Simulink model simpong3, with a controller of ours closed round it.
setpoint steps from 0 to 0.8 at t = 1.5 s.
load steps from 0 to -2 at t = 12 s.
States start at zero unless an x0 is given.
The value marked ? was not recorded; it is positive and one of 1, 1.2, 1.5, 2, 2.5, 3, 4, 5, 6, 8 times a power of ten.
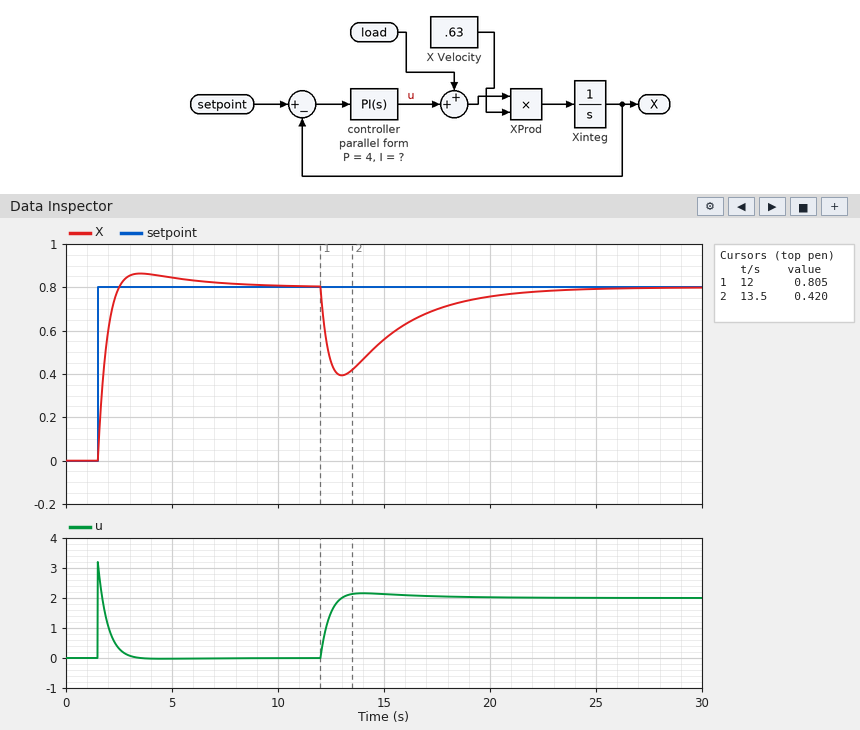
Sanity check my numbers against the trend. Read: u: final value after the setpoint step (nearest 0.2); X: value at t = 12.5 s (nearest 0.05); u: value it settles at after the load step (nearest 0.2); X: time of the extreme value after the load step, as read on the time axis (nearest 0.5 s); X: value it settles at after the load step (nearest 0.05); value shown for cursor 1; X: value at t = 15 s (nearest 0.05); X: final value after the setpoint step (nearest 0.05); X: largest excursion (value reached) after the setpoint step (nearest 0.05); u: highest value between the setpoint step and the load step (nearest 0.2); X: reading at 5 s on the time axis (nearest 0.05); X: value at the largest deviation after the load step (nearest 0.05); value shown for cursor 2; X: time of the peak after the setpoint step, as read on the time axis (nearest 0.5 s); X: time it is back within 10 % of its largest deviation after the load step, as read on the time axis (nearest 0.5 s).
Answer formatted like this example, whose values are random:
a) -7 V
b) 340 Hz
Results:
a) 0.0
b) 0.45
c) 2.0
d) 13.0 s
e) 0.80
f) 0.805
g) 0.55
h) 0.80
i) 0.85
j) 3.2
k) 0.85
l) 0.40
m) 0.420
n) 3.5 s
o) 20.0 s
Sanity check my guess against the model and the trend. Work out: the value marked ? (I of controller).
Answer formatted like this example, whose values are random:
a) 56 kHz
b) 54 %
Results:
a) 1.2
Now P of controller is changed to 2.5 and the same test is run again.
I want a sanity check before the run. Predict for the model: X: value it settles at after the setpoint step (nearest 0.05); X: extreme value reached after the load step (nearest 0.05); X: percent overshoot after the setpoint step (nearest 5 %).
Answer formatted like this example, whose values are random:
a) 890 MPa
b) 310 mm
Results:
a) 0.80
b) 0.25
c) 15 %
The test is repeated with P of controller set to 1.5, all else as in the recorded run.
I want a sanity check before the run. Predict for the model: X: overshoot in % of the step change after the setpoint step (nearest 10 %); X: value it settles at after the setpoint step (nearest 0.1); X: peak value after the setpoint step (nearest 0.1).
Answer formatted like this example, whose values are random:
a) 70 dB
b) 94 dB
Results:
a) 30 %
b) 0.8
c) 1.0
